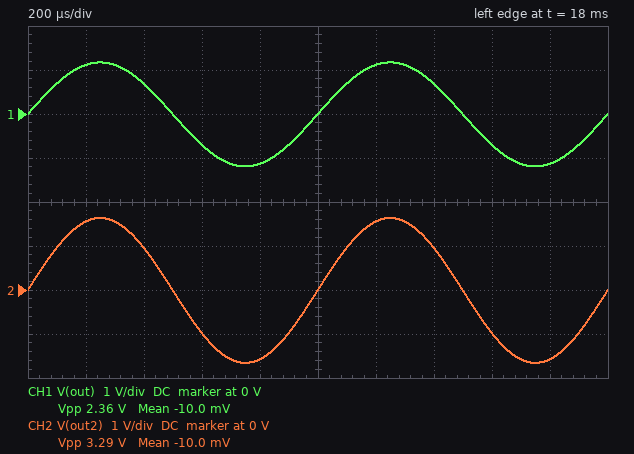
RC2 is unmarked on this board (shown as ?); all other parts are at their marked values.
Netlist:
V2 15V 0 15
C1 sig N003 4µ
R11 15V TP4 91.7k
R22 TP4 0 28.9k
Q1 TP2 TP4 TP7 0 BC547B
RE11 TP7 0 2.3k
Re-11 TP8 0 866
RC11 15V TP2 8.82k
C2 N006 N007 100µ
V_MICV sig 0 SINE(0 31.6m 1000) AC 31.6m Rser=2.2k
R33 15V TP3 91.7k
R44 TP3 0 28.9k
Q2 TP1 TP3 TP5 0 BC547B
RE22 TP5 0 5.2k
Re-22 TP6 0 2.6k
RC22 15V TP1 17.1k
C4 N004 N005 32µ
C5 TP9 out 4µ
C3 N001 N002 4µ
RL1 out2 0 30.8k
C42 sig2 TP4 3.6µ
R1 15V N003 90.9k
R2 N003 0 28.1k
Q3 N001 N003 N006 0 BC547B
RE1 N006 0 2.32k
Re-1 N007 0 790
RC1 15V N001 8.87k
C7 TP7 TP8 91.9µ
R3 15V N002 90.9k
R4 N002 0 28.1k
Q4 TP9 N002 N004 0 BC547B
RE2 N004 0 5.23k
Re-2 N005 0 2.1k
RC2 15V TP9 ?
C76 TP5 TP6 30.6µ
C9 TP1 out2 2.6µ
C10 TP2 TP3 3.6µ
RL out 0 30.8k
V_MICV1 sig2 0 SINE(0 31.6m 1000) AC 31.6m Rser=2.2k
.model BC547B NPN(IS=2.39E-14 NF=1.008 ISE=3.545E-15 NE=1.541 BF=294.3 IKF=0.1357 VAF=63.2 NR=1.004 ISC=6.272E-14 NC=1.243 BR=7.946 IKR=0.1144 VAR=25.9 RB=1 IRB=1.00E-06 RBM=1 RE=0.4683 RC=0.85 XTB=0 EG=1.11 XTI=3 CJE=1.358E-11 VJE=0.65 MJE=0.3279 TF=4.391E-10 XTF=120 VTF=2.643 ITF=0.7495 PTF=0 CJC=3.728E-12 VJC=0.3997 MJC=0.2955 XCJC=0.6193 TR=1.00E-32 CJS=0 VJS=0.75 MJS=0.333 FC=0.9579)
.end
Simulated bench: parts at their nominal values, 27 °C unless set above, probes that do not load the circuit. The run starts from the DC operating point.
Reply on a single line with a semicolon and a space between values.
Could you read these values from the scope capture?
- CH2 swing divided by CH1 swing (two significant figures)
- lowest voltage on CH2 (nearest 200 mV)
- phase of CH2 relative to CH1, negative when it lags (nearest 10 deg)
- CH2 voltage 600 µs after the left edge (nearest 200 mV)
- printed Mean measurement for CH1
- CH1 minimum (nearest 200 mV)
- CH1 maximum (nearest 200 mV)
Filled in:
1.4; -1.6 V; 0 deg; -1.0 V; -10.0 mV; -1.2 V; 1.2 V
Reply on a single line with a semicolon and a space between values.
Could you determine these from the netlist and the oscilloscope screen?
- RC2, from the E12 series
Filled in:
8.2 kΩ
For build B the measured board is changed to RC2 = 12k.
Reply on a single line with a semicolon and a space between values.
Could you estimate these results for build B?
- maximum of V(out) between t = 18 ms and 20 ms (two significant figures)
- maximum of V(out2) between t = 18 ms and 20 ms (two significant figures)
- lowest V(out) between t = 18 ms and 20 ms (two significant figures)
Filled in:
1.6 V; 1.6 V; -1.6 V
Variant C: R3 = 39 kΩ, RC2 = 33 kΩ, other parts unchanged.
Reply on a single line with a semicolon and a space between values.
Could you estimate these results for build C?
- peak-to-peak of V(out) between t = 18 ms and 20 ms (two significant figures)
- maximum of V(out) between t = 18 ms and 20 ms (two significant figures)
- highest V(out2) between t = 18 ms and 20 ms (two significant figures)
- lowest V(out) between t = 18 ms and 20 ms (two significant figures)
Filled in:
98 mV; 49 mV; 1.6 V; -48 mV
